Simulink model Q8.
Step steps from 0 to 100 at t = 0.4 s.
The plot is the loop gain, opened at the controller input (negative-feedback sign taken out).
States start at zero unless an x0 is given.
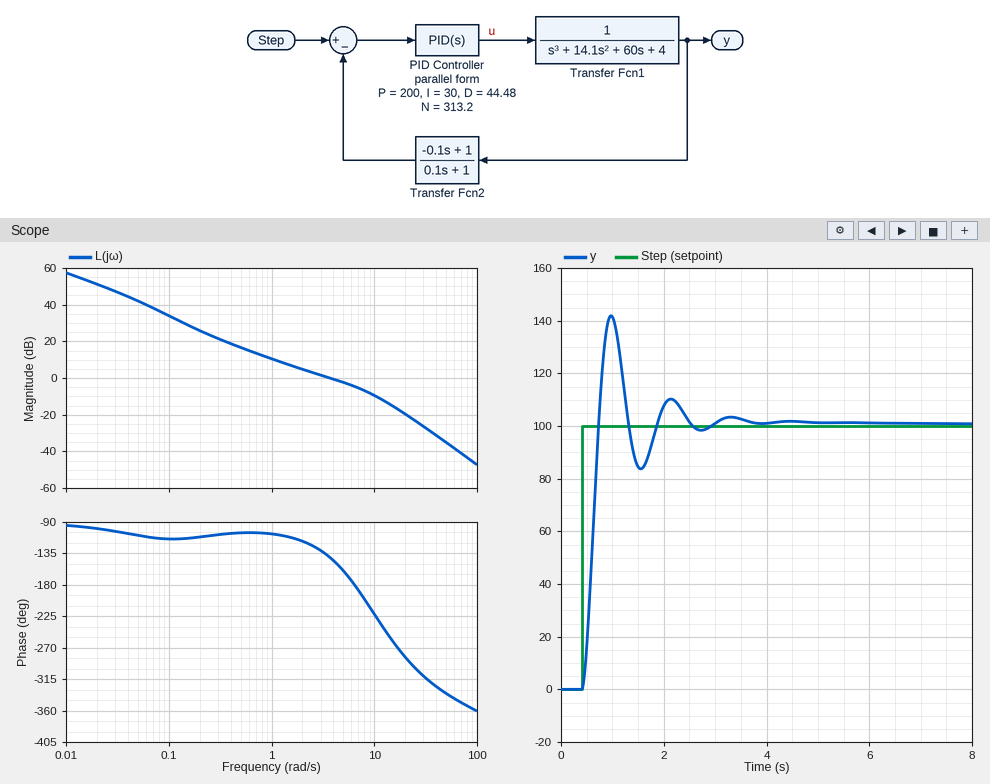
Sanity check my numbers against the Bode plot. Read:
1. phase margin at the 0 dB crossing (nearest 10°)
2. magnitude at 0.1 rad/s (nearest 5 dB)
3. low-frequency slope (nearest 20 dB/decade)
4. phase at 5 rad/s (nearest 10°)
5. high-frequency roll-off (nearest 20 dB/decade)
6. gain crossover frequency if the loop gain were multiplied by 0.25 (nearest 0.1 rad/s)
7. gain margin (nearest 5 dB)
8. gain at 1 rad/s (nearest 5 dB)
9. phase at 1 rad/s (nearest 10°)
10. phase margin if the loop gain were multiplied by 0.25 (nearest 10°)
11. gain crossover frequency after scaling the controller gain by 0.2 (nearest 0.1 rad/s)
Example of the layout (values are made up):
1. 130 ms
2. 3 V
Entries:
1. 40°
2. 35 dB
3. -20 dB/decade
4. -160°
5. -40 dB/decade
6. 0.8 rad/s
7. 5 dB
8. 10 dB
9. -110°
10. 70°
11. 0.7 rad/s
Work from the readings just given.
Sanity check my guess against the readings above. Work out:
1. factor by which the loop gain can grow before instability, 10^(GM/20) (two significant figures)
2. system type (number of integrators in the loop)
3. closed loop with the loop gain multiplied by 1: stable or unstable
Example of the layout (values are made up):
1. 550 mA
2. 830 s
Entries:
1. 1.8
2. 1
3. stable
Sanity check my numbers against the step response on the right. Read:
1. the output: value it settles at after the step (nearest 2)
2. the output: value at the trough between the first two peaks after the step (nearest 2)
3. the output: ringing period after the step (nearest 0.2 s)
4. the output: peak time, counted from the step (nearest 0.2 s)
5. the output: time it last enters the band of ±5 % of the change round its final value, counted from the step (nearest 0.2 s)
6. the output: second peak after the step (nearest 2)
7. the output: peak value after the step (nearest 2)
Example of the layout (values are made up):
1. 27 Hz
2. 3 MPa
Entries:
1. 100
2. 84
3. 1.2 s
4. 0.6 s
5. 2.0 s
6. 110
7. 142
